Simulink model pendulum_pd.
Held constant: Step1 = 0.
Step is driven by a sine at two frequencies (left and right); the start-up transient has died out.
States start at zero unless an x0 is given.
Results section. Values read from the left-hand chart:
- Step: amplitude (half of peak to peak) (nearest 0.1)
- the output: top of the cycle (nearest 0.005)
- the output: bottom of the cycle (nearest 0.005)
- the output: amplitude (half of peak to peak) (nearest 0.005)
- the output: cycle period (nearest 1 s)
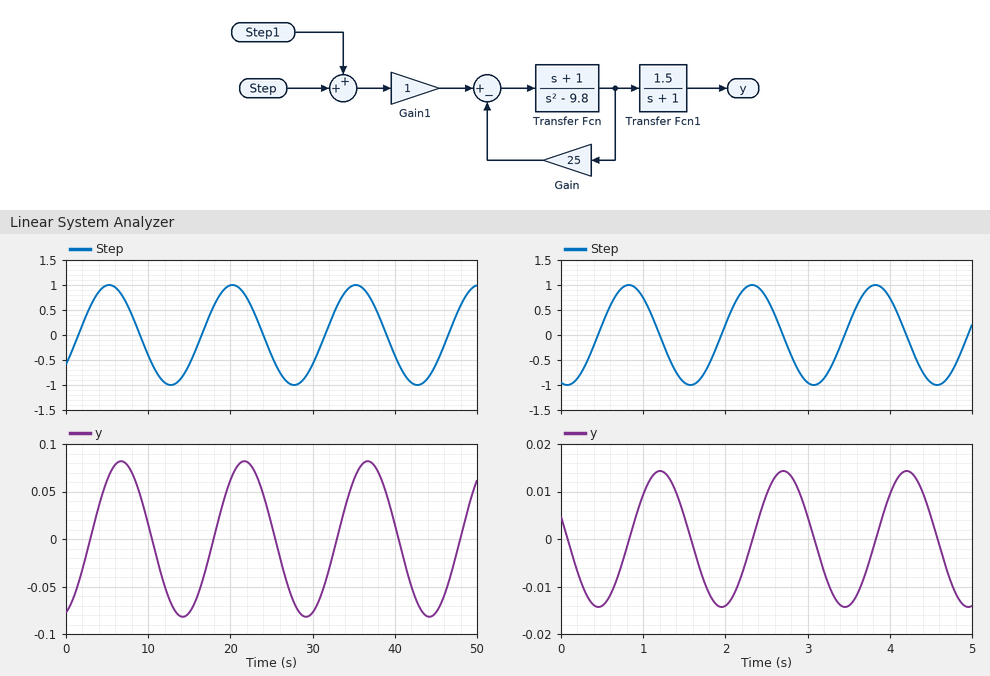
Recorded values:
1.0
0.080
-0.080
0.080
15 s
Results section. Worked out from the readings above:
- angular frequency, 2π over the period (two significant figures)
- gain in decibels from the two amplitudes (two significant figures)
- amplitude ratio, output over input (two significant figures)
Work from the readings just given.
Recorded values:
0.42 rad/s
-22 dB
0.080
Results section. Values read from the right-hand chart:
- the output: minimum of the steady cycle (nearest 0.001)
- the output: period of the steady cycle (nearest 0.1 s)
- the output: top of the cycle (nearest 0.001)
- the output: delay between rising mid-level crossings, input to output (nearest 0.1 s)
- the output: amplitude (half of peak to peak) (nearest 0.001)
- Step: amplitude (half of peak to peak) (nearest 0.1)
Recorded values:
-0.014
1.5 s
0.014
0.4 s
0.014
1.0
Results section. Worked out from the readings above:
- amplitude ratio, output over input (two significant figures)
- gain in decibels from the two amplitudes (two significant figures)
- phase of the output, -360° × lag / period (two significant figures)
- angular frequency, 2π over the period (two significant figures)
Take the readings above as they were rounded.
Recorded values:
0.014
-37 dB
-96°
4.2 rad/s
